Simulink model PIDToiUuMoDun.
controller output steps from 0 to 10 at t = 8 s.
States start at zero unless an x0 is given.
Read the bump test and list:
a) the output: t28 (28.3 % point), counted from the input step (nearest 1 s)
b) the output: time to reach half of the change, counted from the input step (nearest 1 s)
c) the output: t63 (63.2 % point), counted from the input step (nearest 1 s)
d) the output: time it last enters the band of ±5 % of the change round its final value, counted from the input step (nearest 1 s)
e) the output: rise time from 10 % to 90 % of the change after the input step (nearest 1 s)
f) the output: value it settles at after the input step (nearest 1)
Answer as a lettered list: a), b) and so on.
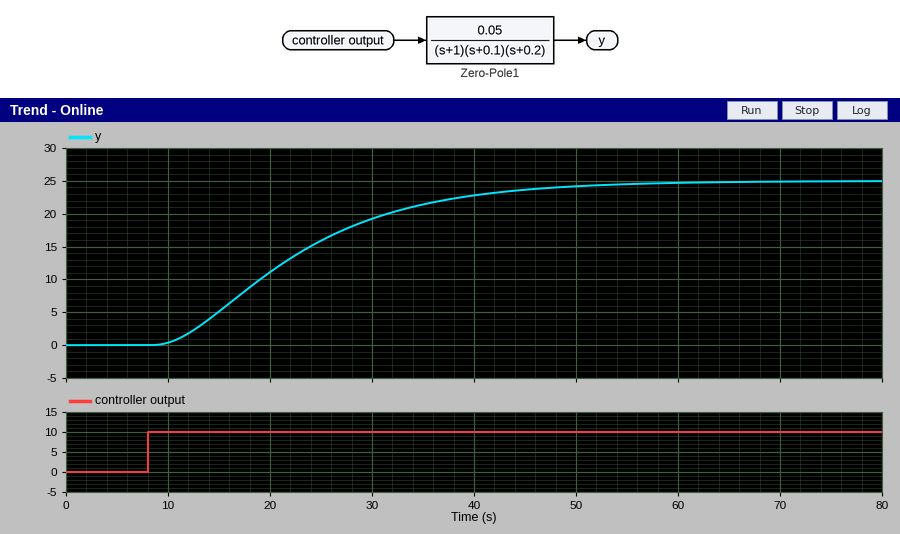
a) 9 s
b) 13 s
c) 17 s
d) 38 s
e) 26 s
f) 25
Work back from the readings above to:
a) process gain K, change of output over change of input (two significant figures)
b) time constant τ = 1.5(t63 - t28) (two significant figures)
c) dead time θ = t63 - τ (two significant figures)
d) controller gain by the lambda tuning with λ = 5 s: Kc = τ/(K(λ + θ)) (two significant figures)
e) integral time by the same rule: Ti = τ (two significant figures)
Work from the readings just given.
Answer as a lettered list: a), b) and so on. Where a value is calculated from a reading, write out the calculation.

a) (25 - 0) / 10 = 2.5
b) 1.5 × (17 - 9) = 12 s
c) 17 - 12 = 5.0 s
d) 12 / (2.5 × (5 + 5)) = 0.48
e) 12 s
